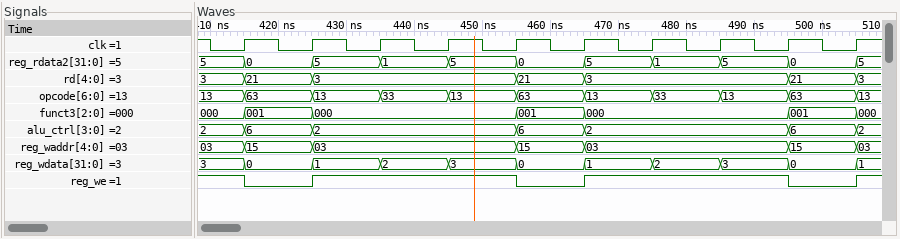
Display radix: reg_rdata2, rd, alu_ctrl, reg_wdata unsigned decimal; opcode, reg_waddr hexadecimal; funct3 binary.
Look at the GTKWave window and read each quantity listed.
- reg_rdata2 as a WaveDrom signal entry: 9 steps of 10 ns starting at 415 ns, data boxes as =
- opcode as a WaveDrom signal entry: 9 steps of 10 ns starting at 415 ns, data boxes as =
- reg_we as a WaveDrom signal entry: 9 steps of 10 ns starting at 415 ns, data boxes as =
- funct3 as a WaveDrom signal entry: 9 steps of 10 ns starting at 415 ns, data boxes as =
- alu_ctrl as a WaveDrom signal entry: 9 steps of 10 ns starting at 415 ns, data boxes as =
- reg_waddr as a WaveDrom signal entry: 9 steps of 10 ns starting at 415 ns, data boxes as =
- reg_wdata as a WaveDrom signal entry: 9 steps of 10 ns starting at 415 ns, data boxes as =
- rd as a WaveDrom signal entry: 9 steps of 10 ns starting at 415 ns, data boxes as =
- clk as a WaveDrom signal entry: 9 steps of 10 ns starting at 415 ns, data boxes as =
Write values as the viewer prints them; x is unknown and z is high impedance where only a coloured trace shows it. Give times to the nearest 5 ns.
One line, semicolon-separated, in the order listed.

{name: 'reg_rdata2', wave: '=========', data: '0 5 1 5 0 5 1 5 0'}; {name: 'opcode', wave: '=========', data: '63 13 33 13 63 13 33 13 63'}; {name: 'reg_we', wave: '01..01..0'}; {name: 'funct3', wave: '==..==..=', data: '001 000 001 000 001'}; {name: 'alu_ctrl', wave: '==..==..=', data: '6 2 6 2 6'}; {name: 'reg_waddr', wave: '==..==..=', data: '15 03 15 03 15'}; {name: 'reg_wdata', wave: '=========', data: '0 1 2 3 0 1 2 3 0'}; {name: 'rd', wave: '==..==..=', data: '21 3 21 3 21'}; {name: 'clk', wave: 'p........'}
